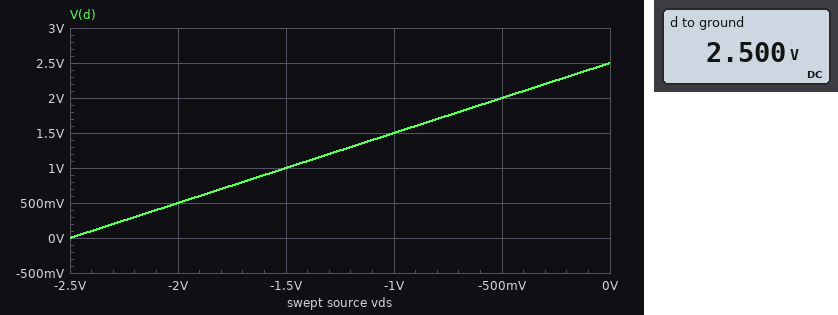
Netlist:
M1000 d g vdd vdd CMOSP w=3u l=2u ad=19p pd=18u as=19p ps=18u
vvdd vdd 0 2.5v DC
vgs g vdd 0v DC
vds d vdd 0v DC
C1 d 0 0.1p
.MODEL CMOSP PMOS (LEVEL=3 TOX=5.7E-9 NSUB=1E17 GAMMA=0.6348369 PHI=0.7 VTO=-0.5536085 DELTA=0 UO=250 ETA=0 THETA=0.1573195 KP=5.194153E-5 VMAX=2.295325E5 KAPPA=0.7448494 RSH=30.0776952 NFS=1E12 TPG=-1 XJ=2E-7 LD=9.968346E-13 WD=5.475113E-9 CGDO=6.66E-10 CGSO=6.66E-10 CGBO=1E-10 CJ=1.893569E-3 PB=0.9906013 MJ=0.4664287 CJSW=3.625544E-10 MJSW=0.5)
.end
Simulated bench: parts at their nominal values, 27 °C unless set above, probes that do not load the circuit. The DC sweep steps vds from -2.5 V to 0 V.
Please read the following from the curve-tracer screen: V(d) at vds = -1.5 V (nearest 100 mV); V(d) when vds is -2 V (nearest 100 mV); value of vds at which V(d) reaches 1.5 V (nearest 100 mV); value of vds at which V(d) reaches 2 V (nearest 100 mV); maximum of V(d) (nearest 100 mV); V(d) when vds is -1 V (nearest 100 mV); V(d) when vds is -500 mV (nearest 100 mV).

1.0 V
500 mV
-1.0 V
-500 mV
2.5 V
1.5 V
2.0 V
